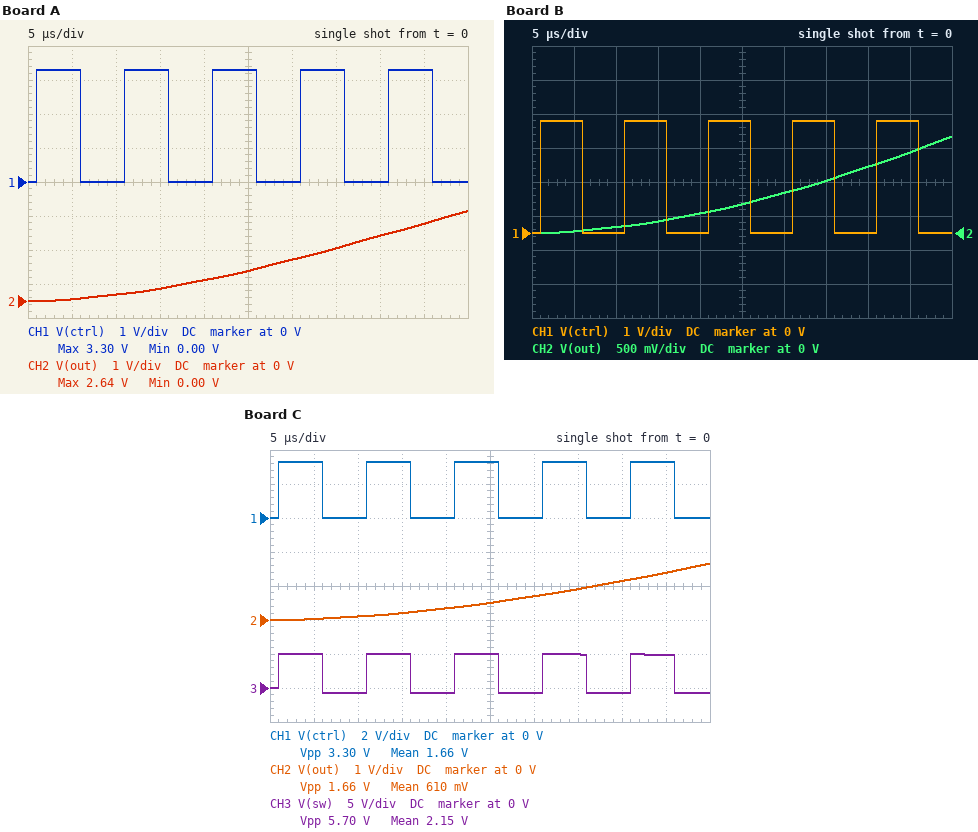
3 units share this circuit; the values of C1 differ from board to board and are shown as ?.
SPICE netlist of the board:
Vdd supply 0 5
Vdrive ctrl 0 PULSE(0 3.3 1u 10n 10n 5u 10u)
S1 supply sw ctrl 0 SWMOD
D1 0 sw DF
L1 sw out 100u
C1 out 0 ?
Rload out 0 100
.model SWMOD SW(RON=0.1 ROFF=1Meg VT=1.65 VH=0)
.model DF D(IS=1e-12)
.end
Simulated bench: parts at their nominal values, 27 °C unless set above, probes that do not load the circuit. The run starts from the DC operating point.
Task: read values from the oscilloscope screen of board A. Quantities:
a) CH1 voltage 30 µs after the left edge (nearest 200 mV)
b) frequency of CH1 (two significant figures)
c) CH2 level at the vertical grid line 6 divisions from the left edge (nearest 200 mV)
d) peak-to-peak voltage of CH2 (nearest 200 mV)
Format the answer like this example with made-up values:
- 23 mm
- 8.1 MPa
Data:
- 0 V
- 100 kHz
- 1.2 V
- 2.6 V
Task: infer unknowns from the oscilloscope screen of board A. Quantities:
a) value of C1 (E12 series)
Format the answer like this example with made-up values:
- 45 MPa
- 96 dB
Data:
- 8.2 µF
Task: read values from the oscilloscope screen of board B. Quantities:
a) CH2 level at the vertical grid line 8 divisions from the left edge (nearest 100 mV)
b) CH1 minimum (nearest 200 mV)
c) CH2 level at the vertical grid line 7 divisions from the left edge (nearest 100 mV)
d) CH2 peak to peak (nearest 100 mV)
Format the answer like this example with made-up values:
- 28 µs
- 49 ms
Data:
- 1.0 V
- 0 V
- 800 mV
- 1.4 V
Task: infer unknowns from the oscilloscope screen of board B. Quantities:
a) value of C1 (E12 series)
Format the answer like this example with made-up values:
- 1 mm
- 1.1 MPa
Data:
- 18 µF
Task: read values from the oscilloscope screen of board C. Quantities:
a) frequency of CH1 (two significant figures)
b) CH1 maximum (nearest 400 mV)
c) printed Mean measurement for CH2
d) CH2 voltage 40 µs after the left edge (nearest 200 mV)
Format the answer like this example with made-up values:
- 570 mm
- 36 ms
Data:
- 100 kHz
- 3.2 V
- 610 mV
- 1.2 V
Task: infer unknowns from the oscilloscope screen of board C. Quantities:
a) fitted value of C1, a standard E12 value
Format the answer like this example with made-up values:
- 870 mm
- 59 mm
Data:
- 15 µF
